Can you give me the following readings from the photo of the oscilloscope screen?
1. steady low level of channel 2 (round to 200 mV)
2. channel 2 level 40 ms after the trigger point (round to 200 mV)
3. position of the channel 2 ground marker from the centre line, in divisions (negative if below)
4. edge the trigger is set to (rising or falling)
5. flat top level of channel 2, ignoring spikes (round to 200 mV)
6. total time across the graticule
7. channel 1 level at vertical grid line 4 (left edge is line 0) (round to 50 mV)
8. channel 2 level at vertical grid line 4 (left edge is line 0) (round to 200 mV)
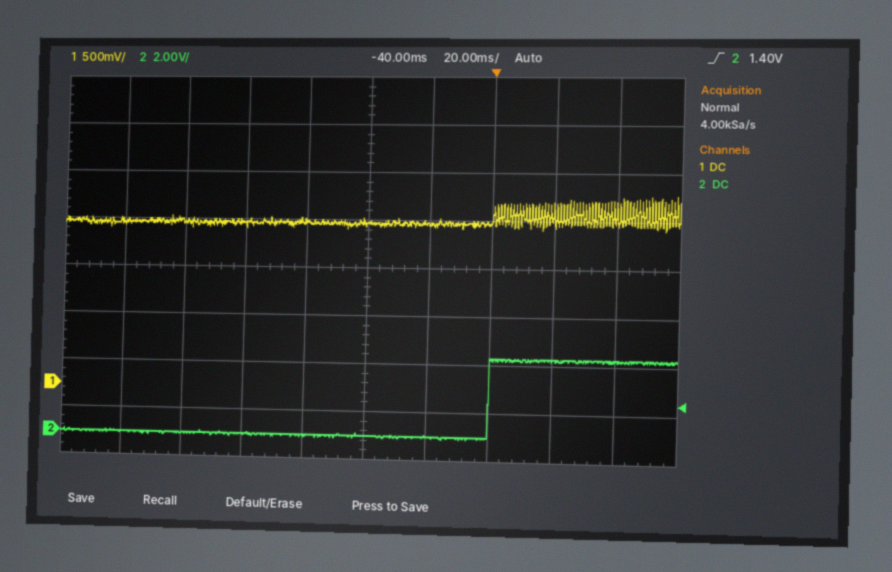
0.0 V
3.2 V
-3.5 div
rising
3.2 V
200 ms
1.75 V
0.0 V
